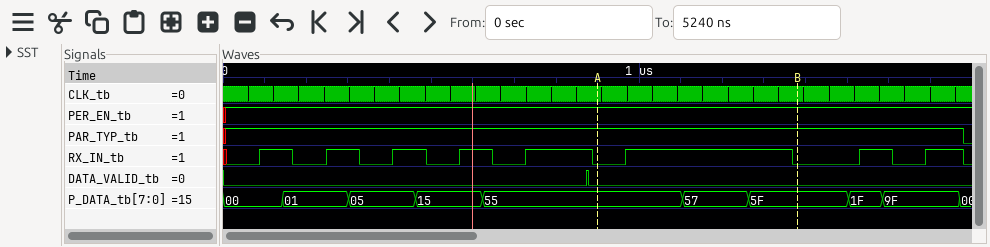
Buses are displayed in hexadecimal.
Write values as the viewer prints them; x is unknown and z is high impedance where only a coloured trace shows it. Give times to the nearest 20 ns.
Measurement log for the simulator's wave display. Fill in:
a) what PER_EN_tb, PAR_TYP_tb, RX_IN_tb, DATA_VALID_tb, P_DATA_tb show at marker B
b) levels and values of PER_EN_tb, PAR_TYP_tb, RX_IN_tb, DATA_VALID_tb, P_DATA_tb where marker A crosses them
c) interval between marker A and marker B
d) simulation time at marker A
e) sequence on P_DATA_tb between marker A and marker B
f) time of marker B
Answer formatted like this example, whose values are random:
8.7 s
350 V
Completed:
PER_EN_tb=1, PAR_TYP_tb=1, RX_IN_tb=0, DATA_VALID_tb=0, P_DATA_tb=5F
PER_EN_tb=1, PAR_TYP_tb=1, RX_IN_tb=0, DATA_VALID_tb=0, P_DATA_tb=55
480 ns
900 ns
55, 57, 5F
1380 ns
